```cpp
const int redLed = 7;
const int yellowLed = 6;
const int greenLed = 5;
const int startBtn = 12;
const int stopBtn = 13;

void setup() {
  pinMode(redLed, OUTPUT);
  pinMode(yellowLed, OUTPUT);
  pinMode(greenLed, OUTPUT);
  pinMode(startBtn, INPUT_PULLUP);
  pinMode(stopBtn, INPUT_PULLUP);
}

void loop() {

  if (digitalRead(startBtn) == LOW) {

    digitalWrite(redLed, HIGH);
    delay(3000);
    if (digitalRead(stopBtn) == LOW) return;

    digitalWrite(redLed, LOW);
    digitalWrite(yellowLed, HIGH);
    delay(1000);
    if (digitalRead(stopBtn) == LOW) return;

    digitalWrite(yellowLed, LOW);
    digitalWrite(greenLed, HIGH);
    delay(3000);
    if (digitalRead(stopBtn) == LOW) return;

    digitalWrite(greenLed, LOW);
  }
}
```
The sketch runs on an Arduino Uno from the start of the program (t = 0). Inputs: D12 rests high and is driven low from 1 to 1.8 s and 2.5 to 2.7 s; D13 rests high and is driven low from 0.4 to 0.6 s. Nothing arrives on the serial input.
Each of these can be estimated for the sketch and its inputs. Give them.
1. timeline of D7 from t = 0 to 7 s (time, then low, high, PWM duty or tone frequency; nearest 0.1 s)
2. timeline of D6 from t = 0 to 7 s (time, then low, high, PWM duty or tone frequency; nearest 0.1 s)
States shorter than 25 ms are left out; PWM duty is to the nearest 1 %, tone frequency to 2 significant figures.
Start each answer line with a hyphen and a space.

- 0 s low; 1 s high; 4 s low
- 0 s low; 4 s high; 5 s low
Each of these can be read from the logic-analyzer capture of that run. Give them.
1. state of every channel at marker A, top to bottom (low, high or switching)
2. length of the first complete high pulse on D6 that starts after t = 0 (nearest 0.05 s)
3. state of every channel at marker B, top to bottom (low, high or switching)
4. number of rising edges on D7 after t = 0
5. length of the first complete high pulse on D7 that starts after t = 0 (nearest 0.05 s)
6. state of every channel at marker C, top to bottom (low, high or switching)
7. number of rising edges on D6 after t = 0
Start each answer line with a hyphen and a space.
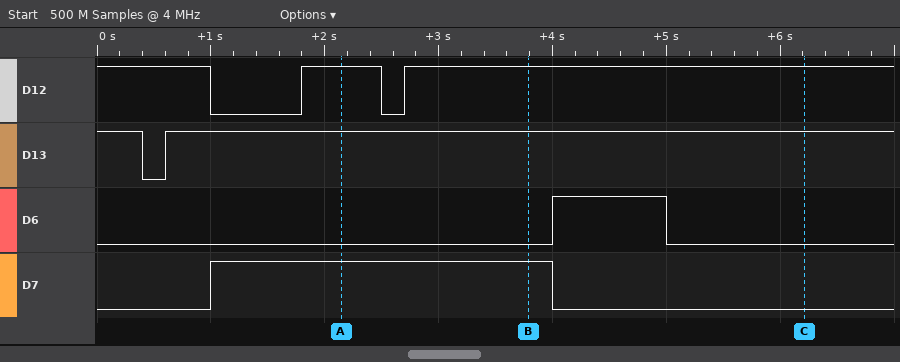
- D12 high, D13 high, D6 low, D7 high
- 1.00 s
- D12 high, D13 high, D6 low, D7 high
- 1
- 3.00 s
- D12 high, D13 high, D6 low, D7 low
- 1
